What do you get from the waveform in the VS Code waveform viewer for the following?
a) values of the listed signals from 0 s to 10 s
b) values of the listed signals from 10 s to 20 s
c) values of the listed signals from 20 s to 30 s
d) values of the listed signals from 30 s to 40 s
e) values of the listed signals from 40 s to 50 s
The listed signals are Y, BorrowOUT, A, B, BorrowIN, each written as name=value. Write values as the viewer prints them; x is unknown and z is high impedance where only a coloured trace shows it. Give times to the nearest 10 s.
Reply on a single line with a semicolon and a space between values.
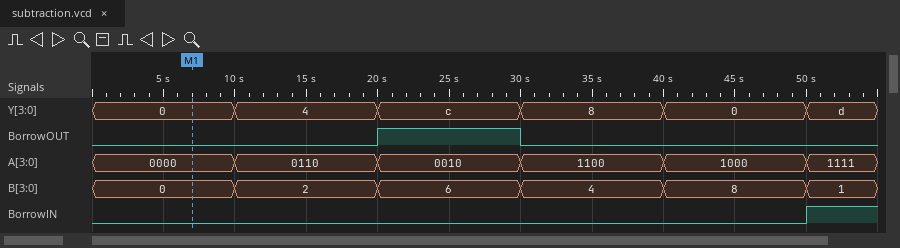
Y=0, BorrowOUT=0, A=0000, B=0, BorrowIN=0; Y=4, BorrowOUT=0, A=0110, B=2, BorrowIN=0; Y=c, BorrowOUT=1, A=0010, B=6, BorrowIN=0; Y=8, BorrowOUT=0, A=1100, B=4, BorrowIN=0; Y=0, BorrowOUT=0, A=1000, B=8, BorrowIN=0
